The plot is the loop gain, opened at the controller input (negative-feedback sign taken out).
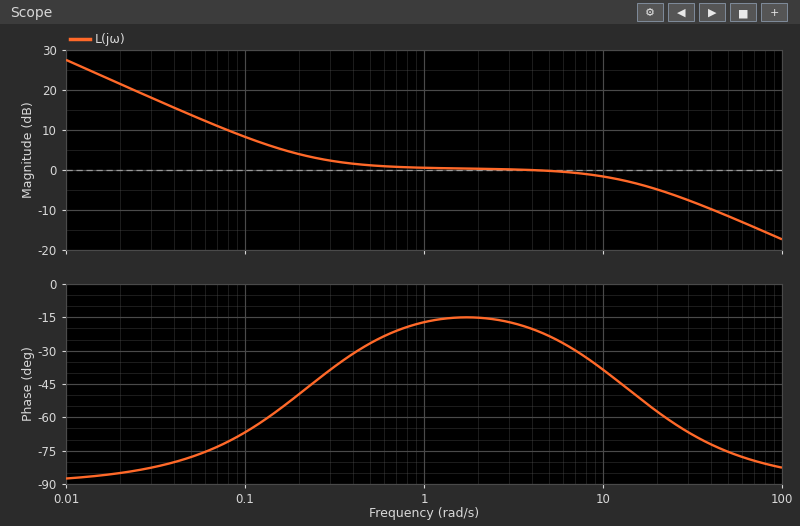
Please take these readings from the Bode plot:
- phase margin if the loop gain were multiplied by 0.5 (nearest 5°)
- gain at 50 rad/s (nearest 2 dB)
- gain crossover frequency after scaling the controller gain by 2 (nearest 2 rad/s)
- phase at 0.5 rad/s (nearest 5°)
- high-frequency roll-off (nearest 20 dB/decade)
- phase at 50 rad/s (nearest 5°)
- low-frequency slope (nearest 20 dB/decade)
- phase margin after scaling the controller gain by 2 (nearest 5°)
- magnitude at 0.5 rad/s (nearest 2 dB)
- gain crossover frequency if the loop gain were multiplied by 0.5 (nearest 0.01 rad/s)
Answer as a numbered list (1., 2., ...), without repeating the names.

1. 120°
2. -12 dB
3. 24 rad/s
4. -25°
5. -20 dB/decade
6. -75°
7. -20 dB/decade
8. 120°
9. 2 dB
10. 0.14 rad/s
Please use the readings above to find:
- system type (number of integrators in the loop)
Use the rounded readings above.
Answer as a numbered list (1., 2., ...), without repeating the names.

1. 1
